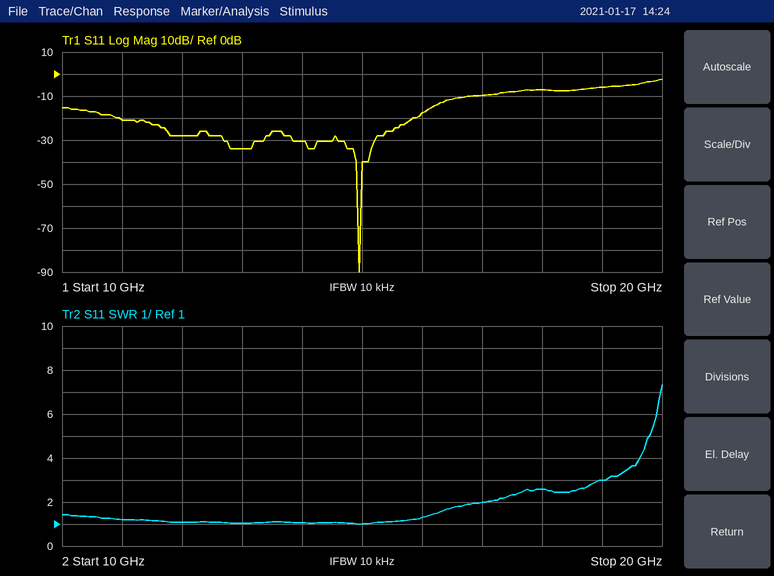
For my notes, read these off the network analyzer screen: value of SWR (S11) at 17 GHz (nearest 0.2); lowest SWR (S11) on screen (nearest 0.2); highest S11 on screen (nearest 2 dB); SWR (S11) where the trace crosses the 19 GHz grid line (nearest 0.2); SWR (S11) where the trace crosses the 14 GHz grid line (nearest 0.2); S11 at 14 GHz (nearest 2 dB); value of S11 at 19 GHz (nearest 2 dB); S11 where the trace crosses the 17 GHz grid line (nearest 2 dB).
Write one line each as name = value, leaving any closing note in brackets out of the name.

value of SWR (S11) at 17 GHz = 2.0
lowest SWR (S11) on screen = 1.0
highest S11 on screen = -2 dB
SWR (S11) where the trace crosses the 19 GHz grid line = 3.0
SWR (S11) where the trace crosses the 14 GHz grid line = 1.0
S11 at 14 GHz = -30 dB
value of S11 at 19 GHz = -6 dB
S11 where the trace crosses the 17 GHz grid line = -10 dB
